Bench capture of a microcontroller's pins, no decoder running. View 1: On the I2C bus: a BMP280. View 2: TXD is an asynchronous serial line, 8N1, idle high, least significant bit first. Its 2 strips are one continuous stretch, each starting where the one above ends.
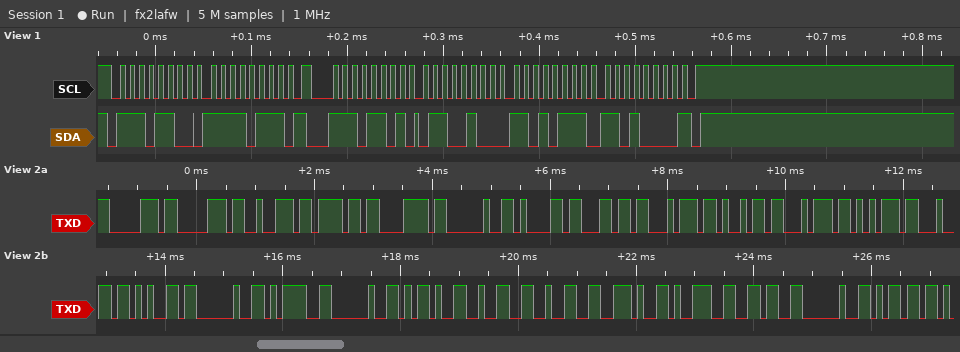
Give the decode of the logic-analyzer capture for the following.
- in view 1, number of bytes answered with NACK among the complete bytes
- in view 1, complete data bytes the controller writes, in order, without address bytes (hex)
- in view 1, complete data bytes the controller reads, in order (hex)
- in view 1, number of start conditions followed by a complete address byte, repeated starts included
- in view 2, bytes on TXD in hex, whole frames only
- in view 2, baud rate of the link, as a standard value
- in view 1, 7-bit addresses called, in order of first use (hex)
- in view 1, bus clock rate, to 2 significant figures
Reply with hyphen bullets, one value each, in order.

- 1
- F7
- 64 D7 D0
- 2
- 0x70 0x70 0x72 0x6F 0x78 0x20 0x61 0x6C 0x74 0x69 0x74 0x75 0x64 0x65 0x20 0x3D 0x20 0x2D 0x32 0x32 0x2E 0x39 0x36 0x20 0x6D
- 9600 baud
- 0x76
- 100 kHz
